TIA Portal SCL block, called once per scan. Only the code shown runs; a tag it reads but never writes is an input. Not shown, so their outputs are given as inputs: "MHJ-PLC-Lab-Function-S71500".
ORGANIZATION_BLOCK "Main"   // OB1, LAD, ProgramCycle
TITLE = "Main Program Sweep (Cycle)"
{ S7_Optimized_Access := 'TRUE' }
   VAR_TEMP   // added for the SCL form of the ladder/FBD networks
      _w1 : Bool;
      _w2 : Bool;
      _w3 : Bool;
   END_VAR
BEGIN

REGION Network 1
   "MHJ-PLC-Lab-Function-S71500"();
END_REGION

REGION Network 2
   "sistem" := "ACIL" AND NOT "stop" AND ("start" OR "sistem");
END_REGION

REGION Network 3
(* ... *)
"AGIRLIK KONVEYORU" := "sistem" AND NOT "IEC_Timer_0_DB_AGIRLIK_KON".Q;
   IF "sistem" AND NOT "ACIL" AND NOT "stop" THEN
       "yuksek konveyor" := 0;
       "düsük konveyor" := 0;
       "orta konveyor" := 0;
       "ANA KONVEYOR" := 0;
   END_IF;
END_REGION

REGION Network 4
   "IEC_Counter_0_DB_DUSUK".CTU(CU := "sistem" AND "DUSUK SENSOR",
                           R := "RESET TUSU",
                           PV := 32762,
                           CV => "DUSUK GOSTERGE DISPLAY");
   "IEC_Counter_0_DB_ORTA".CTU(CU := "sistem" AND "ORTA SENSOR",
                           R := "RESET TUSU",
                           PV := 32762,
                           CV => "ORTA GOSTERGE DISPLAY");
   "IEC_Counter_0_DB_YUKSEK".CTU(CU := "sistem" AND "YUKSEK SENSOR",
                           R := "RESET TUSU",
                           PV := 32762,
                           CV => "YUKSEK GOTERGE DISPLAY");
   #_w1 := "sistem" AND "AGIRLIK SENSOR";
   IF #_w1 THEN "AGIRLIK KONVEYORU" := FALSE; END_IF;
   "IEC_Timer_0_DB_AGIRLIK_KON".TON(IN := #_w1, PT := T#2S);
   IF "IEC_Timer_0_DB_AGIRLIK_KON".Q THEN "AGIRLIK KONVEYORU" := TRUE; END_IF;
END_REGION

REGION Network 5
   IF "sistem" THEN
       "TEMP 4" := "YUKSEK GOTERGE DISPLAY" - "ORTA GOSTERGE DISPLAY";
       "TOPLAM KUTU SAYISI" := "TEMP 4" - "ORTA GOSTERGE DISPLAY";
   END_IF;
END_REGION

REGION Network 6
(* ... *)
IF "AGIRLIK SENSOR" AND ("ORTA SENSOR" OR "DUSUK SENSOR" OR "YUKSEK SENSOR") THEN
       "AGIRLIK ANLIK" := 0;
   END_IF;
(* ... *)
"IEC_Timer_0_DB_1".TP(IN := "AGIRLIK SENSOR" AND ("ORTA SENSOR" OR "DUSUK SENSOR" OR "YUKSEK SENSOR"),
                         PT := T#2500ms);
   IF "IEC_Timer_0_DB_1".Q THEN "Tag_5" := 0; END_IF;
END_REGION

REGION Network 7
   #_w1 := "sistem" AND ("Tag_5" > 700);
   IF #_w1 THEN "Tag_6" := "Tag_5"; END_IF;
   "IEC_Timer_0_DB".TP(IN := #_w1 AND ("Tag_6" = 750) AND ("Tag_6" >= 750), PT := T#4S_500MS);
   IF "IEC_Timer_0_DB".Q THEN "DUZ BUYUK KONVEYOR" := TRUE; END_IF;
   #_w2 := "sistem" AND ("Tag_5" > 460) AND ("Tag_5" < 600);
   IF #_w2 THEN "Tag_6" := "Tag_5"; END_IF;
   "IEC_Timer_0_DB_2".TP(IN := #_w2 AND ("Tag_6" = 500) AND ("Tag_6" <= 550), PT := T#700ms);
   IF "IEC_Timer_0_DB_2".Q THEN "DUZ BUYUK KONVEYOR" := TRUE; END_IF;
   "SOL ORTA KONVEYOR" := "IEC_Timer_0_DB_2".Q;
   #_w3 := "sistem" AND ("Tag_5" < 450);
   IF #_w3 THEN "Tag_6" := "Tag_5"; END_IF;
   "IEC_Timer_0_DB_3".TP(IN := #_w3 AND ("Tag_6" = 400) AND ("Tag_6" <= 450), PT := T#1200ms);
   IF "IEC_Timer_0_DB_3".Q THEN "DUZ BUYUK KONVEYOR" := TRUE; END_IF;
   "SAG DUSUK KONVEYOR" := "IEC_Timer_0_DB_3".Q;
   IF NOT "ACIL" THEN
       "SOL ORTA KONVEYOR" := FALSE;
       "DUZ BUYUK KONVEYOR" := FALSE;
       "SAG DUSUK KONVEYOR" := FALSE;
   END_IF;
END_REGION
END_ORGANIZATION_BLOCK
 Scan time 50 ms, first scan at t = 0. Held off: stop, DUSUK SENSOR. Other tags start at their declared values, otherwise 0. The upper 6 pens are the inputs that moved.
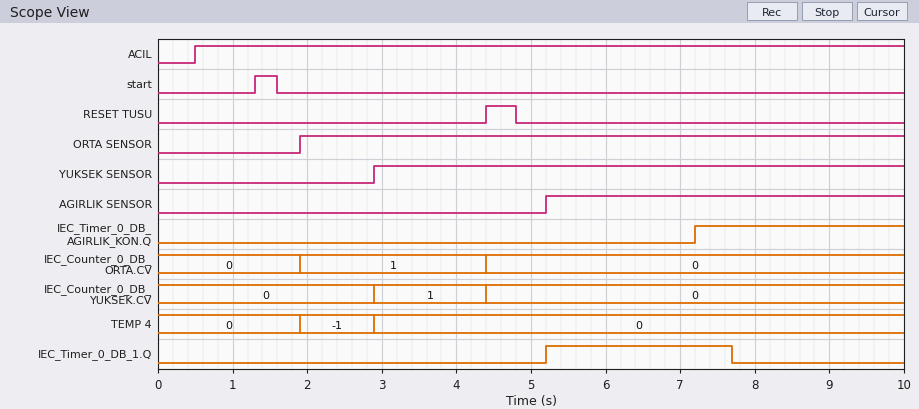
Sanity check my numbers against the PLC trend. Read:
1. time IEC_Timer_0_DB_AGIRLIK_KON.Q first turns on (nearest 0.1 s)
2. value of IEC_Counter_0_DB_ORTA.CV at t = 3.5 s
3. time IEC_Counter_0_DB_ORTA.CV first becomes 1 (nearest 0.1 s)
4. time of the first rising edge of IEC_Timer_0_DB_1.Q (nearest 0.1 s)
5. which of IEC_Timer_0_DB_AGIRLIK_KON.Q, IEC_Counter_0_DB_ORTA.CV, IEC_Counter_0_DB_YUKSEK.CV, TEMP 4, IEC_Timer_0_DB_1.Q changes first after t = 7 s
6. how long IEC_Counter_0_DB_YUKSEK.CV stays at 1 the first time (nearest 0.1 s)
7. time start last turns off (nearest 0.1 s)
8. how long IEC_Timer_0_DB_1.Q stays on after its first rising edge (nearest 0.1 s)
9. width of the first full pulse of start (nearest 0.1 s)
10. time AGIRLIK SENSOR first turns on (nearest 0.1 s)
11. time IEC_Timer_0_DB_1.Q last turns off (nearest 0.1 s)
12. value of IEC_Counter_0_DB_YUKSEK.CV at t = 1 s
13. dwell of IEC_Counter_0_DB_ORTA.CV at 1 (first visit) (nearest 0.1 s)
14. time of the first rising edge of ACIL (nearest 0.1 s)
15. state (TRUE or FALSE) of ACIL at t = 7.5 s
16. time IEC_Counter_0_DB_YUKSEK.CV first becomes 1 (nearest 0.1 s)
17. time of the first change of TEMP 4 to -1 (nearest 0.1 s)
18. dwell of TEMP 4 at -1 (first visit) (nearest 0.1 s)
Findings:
7.2 s
1
1.9 s
5.2 s
IEC_Timer_0_DB_AGIRLIK_KON.Q
1.5 s
1.6 s
2.5 s
0.3 s
5.2 s
7.7 s
0
2.5 s
0.5 s
TRUE
2.9 s
1.9 s
1.0 s
